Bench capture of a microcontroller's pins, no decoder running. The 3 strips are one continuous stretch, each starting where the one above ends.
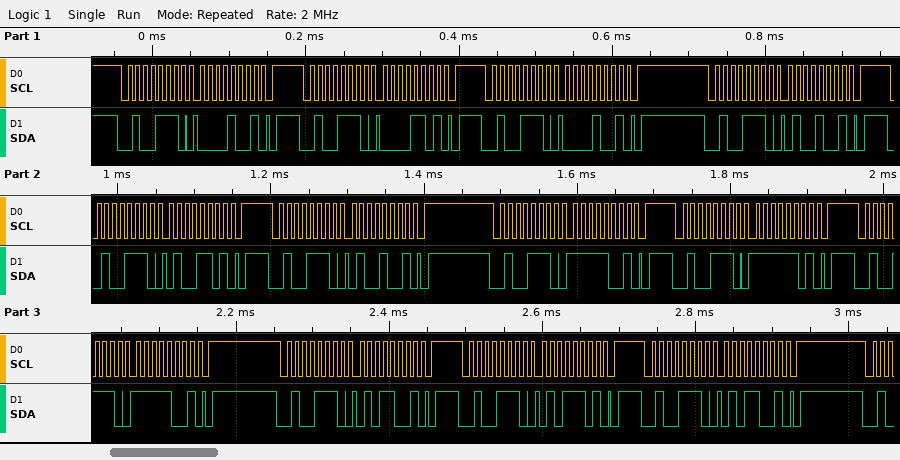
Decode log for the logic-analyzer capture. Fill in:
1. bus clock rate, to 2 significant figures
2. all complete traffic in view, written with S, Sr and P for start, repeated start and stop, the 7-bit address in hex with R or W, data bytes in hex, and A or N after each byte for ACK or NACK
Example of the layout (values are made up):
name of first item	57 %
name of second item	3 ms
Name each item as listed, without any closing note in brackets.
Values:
bus clock rate, to 2 significant figures	100 kHz
all complete traffic in view, written with S, Sr and P for start, repeated start and stop, the 7-bit address in hex with R or W, data bytes in hex, and A or N after each byte for ACK or NACK	S 27W A 09 A P S 27W A 0D A P S 27W A 09 A P S 27W A 49 A P S 27W A 4D A P S 27W A 49 A P S 27W A F9 A P S 27W A FD A P S 27W A F9 A P S 27W A 59 A P S 27W A 5D A P S 27W A 59 A P
